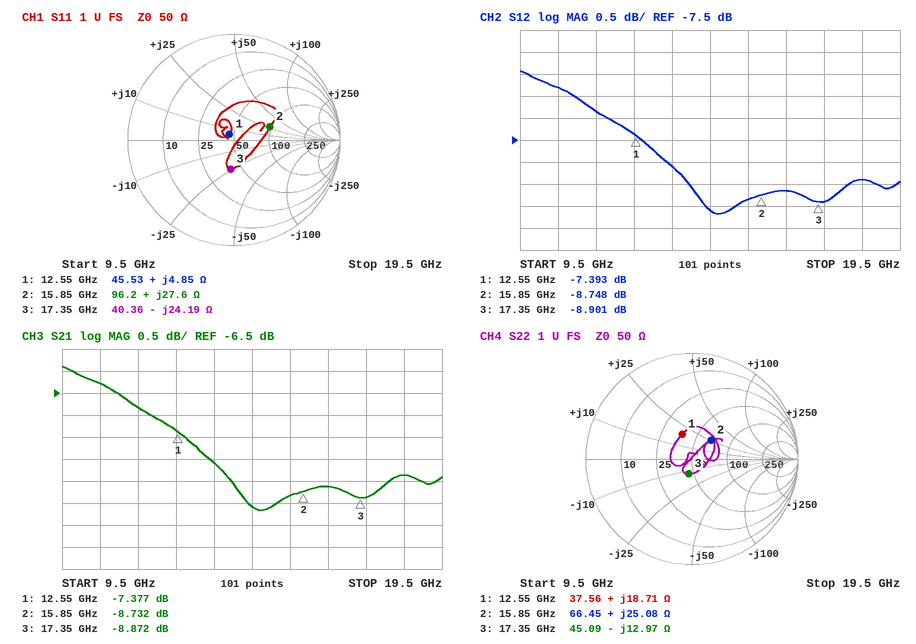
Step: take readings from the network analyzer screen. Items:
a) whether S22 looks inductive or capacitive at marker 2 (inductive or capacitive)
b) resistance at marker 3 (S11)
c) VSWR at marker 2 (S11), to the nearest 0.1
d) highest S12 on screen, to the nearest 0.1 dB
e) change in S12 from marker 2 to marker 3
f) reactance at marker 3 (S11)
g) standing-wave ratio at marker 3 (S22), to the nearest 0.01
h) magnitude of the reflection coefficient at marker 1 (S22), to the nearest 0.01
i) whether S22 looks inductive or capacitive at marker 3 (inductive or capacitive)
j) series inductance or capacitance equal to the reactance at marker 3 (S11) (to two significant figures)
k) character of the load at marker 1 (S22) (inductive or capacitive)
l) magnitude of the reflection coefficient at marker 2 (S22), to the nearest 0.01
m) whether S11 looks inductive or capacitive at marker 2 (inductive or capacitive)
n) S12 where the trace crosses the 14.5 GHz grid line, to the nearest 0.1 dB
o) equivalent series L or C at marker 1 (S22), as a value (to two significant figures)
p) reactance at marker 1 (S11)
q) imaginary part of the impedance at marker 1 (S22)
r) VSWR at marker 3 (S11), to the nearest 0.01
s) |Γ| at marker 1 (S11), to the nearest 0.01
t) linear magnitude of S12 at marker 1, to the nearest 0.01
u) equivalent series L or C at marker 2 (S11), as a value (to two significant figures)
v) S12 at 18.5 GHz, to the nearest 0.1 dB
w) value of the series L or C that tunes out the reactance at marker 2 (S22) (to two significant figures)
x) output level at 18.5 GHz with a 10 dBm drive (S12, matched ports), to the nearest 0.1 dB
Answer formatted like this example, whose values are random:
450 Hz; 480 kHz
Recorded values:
inductive; 40.36 Ω; 2.1; -5.9 dB; -0.153 dB; -24.19 Ω; 1.34; 0.25; capacitive; 380 fF; inductive; 0.25; inductive; -9.1 dB; 240 pH; +4.85 Ω; +18.71 Ω; 1.77; 0.07; 0.43; 280 pH; -8.4 dB; 400 fF; 1.6 dBm
